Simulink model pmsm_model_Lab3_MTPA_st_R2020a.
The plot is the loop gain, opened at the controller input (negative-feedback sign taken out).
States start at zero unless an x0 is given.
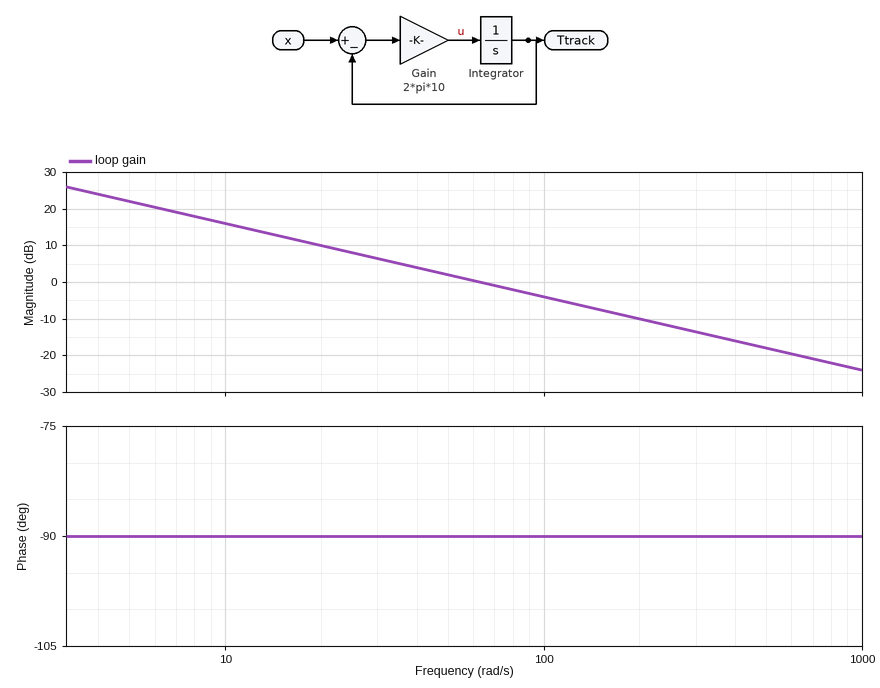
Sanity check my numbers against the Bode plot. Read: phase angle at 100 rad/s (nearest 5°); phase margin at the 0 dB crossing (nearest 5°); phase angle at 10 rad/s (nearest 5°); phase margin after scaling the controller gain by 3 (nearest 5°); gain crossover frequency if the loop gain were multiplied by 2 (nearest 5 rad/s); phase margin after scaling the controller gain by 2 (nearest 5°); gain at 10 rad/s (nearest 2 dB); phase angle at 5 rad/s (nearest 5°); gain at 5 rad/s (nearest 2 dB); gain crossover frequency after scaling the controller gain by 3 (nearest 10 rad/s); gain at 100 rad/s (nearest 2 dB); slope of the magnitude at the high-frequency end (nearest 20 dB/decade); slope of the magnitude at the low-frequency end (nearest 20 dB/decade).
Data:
-90°
90°
-90°
90°
125 rad/s
90°
16 dB
-90°
22 dB
190 rad/s
-4 dB
-20 dB/decade
-20 dB/decade
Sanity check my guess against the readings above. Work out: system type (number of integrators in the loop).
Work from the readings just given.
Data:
1
